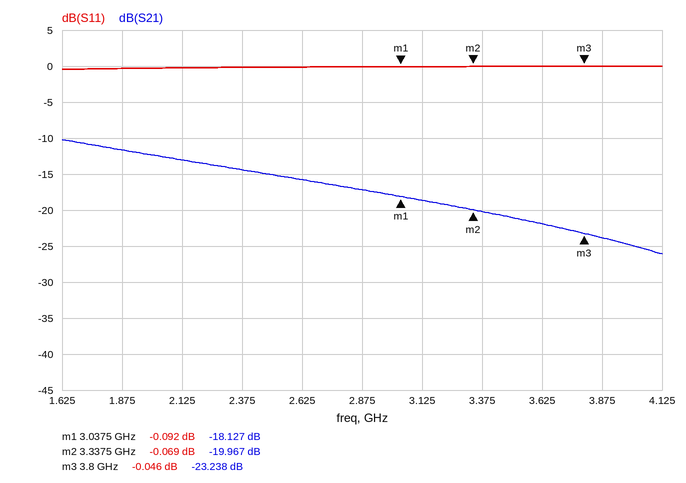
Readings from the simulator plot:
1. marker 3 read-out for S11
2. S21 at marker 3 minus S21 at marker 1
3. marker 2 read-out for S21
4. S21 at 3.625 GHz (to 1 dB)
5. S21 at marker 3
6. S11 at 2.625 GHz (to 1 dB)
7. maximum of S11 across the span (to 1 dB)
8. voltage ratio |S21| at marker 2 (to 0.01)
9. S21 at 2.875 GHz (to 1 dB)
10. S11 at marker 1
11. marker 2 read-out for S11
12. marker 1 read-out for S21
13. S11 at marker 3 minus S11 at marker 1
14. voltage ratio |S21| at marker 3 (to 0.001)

-0.046 dB
-5.111 dB
-19.967 dB
-22 dB
-23.238 dB
0 dB
0 dB
0.10
-17 dB
-0.092 dB
-0.069 dB
-18.127 dB
0.046 dB
0.069
